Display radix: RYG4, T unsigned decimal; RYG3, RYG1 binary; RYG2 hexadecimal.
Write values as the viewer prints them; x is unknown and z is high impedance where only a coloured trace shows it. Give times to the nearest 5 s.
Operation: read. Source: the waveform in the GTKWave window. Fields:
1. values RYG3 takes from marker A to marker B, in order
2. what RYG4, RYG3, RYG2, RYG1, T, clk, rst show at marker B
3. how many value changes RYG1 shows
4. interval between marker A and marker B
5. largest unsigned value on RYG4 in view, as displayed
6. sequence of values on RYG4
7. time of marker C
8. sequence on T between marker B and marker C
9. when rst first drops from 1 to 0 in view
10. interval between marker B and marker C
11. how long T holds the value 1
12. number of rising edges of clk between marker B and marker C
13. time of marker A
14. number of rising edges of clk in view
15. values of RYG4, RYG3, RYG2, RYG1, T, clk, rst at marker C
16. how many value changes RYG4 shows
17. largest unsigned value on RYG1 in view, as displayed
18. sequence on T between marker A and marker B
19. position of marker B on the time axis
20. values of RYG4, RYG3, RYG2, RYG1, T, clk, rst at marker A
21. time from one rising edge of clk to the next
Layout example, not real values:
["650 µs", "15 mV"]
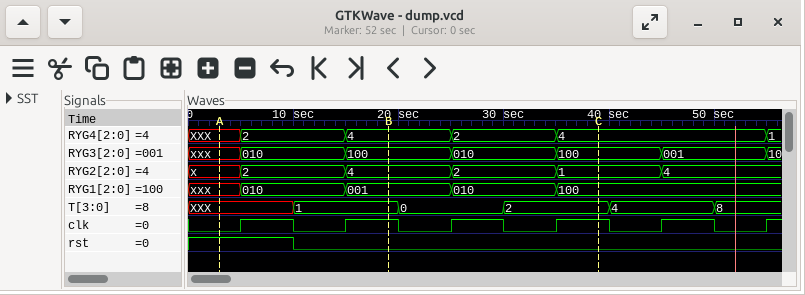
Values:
["xxx, 010, 100", "RYG4=4, RYG3=100, RYG2=4, RYG1=001, T=1, clk=1, rst=0", "4", "15 s", "4", "XXX, 2, 4, 2, 4, 1", "40 s", "1, 0, 2", "10 s", "20 s", "10 s", "2", "5 s", "6", "RYG4=4, RYG3=100, RYG2=1, RYG1=100, T=2, clk=1, rst=0", "5", "100", "XXX, 1", "20 s", "RYG4=XXX, RYG3=xxx, RYG2=x, RYG1=xxx, T=XXX, clk=0, rst=1", "10 s"]
